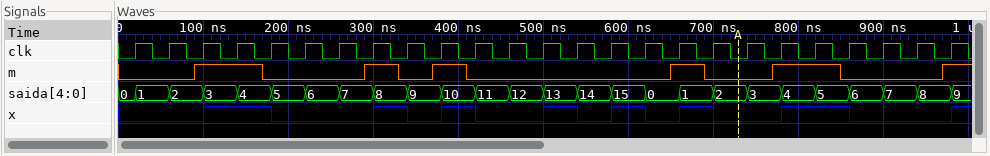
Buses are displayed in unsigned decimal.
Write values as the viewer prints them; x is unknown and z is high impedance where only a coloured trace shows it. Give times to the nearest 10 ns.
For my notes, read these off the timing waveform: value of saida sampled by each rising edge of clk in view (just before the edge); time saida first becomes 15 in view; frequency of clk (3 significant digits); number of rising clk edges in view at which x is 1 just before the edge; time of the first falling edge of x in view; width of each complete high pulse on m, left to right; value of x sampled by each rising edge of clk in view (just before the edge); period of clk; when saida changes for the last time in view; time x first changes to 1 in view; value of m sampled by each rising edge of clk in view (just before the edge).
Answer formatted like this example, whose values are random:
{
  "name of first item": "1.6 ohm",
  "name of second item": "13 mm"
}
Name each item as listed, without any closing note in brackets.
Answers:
{
  "value of saida sampled by each rising edge of clk in view": "0, 1, 2, 3, 4, 5, 6, 7, 8, 9, 10, 11, 12, 13, 14, 15, 0, 1, 2, 3, 4, 5, 6, 7, 8",
  "time saida first becomes 15 in view": "580 ns",
  "frequency of clk": "25.0 MHz",
  "number of rising clk edges in view at which x is 1 just before the edge": "9",
  "time of the first falling edge of x in view": "180 ns",
  "width of each complete high pulse on m, left to right": "80 ns, 40 ns, 40 ns, 40 ns, 80 ns",
  "value of x sampled by each rising edge of clk in view": "0 0 0 1 1 0 0 0 1 0 1 0 0 1 0 1 0 1 0 0 1 1 0 0 0",
  "period of clk": "40 ns",
  "when saida changes for the last time in view": "980 ns",
  "time x first changes to 1 in view": "100 ns",
  "value of m sampled by each rising edge of clk in view": "0 0 1 1 0 0 0 1 0 1 0 0 0 0 0 0 1 0 0 1 1 0 0 0 1"
}
